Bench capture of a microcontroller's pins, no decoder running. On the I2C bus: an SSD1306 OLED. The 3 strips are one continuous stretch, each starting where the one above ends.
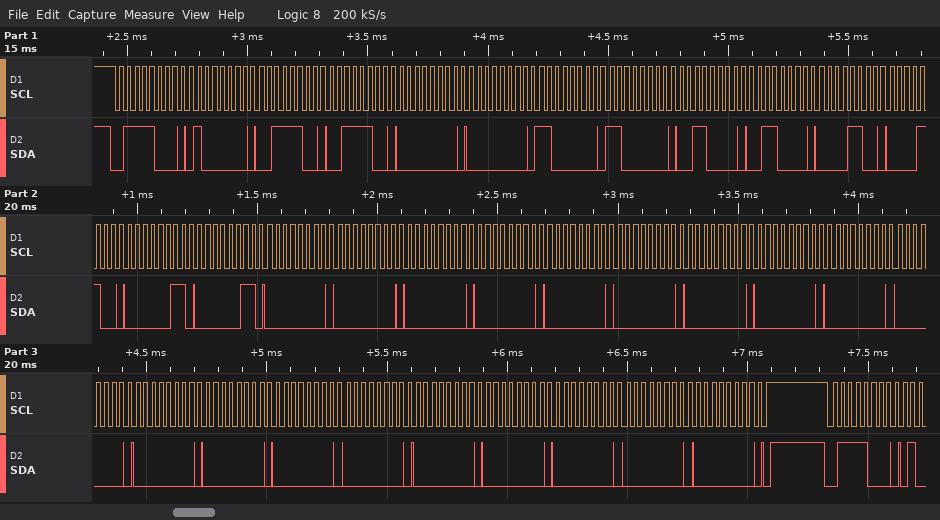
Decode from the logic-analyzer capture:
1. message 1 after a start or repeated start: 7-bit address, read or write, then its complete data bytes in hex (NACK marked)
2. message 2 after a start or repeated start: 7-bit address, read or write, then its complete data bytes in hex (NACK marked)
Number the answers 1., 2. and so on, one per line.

1. 0x3C write: 40 3C 3C 00 00 C0 C0 30 30 0C 0C 03 03 00 00 00 00 00 00 00 00 00 00 00 00 00 00 00 00 00 00 00
2. 0x3C write
